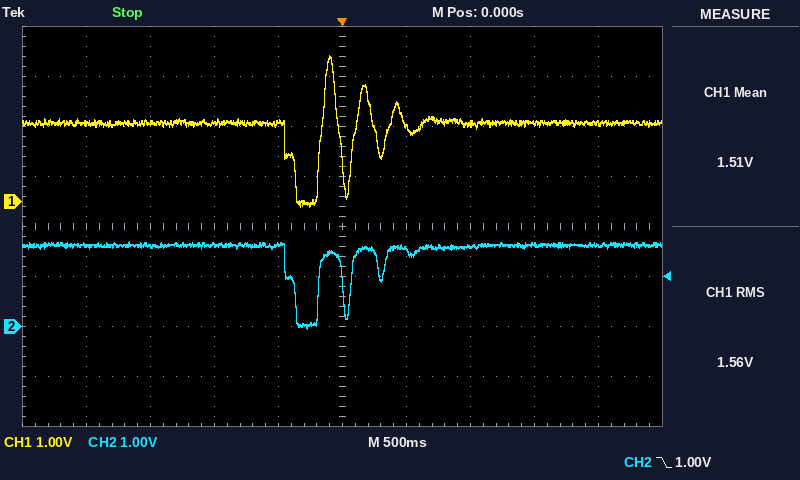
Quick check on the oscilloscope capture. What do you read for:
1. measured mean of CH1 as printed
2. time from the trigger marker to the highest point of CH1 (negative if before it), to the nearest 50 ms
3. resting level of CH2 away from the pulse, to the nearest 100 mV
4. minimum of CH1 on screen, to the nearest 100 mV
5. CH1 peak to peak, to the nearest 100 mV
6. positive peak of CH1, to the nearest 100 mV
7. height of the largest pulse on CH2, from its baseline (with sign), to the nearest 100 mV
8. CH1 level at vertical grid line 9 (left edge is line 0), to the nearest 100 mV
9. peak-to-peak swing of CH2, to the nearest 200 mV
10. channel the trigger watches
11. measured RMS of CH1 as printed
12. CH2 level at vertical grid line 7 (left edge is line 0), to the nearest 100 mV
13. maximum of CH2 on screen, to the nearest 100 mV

1.51 V
-100 ms
1.6 V
-100 mV
3.0 V
2.9 V
-1.7 V
1.6 V
1.8 V
CH2
1.56 V
1.6 V
1.7 V
